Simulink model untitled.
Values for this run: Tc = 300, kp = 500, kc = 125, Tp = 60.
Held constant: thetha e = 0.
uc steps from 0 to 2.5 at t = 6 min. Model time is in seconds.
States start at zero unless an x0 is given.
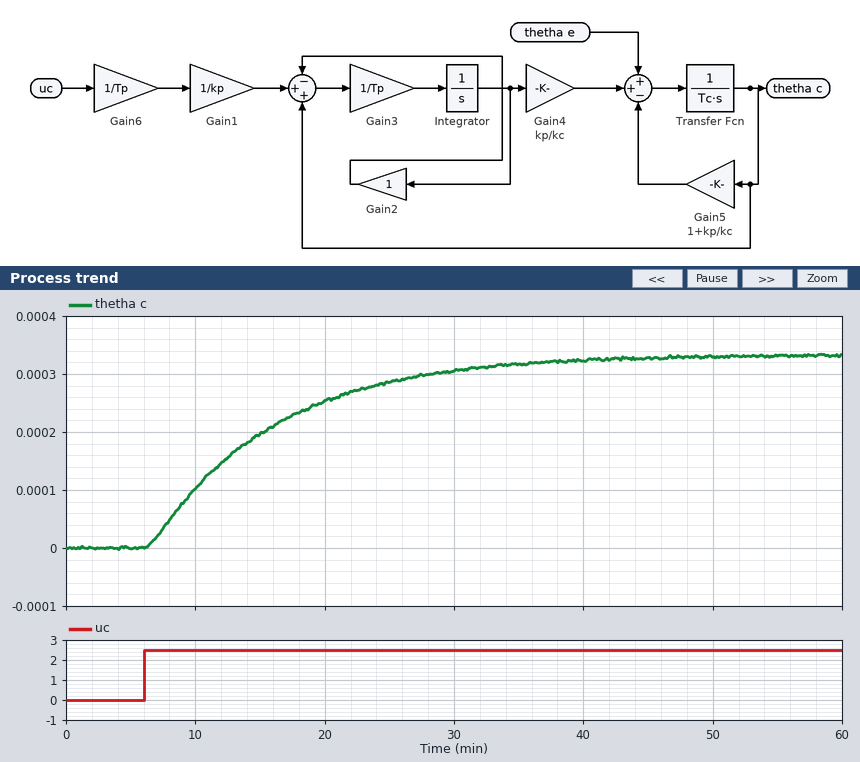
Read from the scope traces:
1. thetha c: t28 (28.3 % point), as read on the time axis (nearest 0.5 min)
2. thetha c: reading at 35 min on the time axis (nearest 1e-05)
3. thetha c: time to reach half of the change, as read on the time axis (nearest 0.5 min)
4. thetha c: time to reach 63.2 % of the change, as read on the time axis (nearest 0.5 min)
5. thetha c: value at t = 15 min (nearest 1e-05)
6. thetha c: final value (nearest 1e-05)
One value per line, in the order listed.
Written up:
9.5 min
0.00032
13.0 min
16.0 min
0.00020
0.00033
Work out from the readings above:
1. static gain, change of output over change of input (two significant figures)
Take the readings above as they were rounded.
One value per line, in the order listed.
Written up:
0.00013
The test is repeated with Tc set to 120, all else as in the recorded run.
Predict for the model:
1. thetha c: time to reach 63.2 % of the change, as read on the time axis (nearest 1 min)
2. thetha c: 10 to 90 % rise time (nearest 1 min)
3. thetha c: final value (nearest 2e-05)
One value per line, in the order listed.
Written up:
13 min
15 min
0.00034
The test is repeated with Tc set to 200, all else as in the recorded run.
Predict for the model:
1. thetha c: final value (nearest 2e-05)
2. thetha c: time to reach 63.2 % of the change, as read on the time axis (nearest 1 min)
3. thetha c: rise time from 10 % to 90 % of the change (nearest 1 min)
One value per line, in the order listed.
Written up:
0.00034
14 min
17 min
